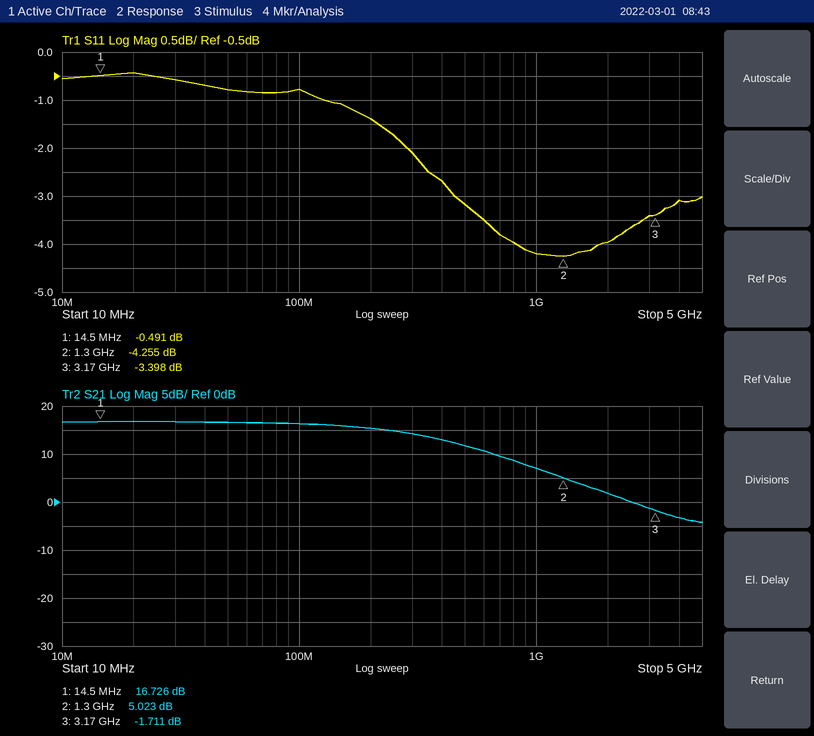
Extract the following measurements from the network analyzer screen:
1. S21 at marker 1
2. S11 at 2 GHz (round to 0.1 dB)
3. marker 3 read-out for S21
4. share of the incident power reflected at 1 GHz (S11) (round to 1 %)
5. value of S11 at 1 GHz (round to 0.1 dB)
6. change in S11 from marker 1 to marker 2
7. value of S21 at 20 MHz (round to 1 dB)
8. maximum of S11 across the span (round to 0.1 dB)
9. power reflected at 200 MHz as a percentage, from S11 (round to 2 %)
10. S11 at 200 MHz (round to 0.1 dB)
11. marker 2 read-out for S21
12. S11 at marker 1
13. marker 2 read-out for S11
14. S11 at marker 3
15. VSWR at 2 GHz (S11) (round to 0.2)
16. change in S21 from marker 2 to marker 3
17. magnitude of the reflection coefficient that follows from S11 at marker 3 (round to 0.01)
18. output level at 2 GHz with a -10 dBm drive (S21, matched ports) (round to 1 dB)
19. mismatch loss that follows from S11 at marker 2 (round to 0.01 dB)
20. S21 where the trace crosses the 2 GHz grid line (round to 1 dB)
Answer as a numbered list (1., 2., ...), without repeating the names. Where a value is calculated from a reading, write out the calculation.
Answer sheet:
1. 16.726 dB
2. -4.0 dB
3. -1.711 dB
4. 10^(-4.2/10) ≈ 38 %
5. -4.2 dB
6. -4.255 − (-0.491) = -3.764 dB
7. 17 dB
8. -0.4 dB
9. 10^(-1.4/10) ≈ 72 %
10. -1.4 dB
11. 5.023 dB
12. -0.491 dB
13. -4.255 dB
14. -3.398 dB
15. |Γ| = 10^(-4/20) = 0.6310; VSWR = (1 + 0.6310)/(1 − 0.6310) ≈ 4.4
16. -1.711 − (5.023) = -6.734 dB
17. 10^(-3.398/20) ≈ 0.68
18. -10 dBm + (2 dB) = -8 dBm
19. −10 log10(1 − 10^(-4.255/10)) ≈ 2.04 dB
20. 2 dB
